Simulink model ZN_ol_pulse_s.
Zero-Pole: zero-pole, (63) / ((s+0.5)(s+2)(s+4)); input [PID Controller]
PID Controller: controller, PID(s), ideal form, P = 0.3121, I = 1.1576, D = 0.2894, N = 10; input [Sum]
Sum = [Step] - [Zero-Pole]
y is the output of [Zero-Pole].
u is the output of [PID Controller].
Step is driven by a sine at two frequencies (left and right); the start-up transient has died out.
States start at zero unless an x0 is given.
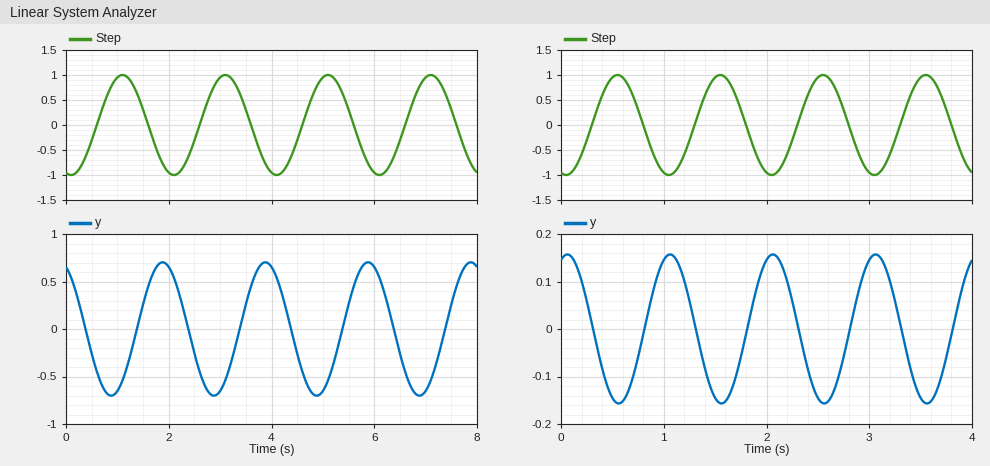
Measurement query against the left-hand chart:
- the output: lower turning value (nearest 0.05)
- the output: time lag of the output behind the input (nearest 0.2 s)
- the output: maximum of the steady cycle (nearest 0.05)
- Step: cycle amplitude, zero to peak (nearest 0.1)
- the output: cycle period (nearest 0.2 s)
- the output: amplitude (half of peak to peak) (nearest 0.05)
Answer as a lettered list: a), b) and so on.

a) -0.70
b) 0.8 s
c) 0.70
d) 1.0
e) 2.0 s
f) 0.70
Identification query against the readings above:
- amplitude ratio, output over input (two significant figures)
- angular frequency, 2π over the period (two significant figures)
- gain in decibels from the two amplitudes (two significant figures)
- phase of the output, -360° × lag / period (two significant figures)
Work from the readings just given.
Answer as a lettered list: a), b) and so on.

a) 0.70
b) 3.1 rad/s
c) -3.1 dB
d) -140°
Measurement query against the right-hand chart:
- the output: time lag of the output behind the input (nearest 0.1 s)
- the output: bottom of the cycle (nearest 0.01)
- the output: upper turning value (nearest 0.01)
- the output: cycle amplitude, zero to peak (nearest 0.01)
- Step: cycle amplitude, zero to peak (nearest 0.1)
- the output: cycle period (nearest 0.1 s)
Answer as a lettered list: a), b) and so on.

a) 0.5 s
b) -0.16
c) 0.16
d) 0.16
e) 1.0
f) 1.0 s
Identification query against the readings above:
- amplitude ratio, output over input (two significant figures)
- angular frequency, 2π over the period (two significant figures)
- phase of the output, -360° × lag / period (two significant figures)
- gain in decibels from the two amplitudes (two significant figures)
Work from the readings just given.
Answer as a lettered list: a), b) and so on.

a) 0.16
b) 6.3 rad/s
c) -180°
d) -16 dB
